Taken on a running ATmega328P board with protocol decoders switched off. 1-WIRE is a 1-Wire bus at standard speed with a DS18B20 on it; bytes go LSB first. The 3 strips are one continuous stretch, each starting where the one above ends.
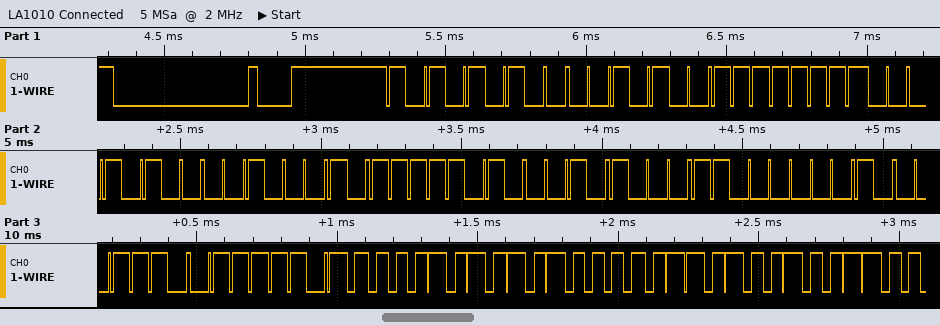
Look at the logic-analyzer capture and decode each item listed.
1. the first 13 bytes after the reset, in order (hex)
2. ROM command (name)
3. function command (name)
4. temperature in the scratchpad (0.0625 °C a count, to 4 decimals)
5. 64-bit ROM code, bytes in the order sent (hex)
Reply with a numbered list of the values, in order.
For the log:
1. 55 28 FF 28 44 5F 14 03 71 BE 50 05 4B
2. Match ROM
3. Read Scratchpad
4. 85.0000 °C
5. 28 FF 28 44 5F 14 03 71
